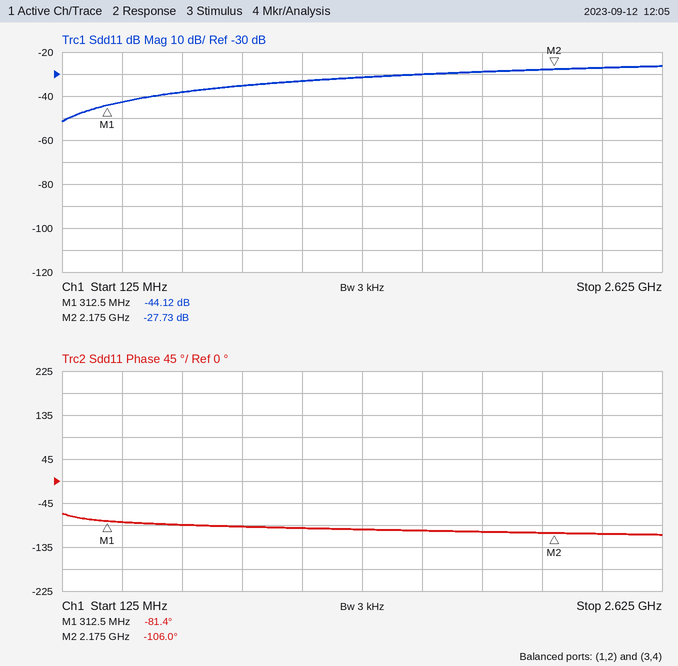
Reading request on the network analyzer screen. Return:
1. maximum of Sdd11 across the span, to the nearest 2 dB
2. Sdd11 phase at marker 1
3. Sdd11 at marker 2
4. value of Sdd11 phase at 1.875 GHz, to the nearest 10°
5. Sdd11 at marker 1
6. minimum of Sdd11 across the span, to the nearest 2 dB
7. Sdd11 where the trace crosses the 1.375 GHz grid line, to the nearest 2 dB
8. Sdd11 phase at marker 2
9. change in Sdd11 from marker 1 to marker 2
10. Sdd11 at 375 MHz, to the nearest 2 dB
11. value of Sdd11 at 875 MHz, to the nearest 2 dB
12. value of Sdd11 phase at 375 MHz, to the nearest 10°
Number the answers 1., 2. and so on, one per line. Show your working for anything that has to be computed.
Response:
1. -26 dB
2. -81.4°
3. -27.73 dB
4. -100°
5. -44.12 dB
6. -52 dB
7. -32 dB
8. -106.0°
9. -27.73 − (-44.12) = 16.39 dB
10. -42 dB
11. -36 dB
12. -80°
